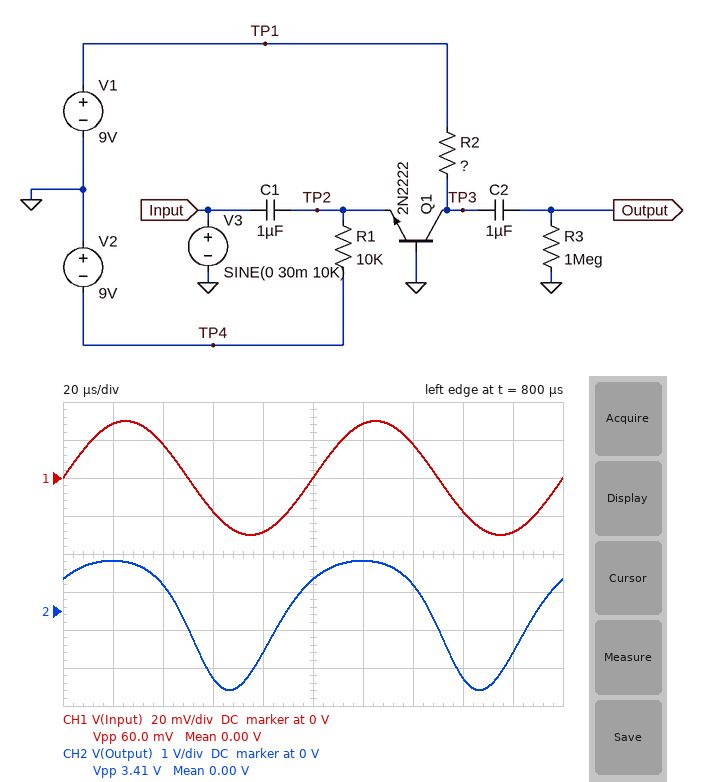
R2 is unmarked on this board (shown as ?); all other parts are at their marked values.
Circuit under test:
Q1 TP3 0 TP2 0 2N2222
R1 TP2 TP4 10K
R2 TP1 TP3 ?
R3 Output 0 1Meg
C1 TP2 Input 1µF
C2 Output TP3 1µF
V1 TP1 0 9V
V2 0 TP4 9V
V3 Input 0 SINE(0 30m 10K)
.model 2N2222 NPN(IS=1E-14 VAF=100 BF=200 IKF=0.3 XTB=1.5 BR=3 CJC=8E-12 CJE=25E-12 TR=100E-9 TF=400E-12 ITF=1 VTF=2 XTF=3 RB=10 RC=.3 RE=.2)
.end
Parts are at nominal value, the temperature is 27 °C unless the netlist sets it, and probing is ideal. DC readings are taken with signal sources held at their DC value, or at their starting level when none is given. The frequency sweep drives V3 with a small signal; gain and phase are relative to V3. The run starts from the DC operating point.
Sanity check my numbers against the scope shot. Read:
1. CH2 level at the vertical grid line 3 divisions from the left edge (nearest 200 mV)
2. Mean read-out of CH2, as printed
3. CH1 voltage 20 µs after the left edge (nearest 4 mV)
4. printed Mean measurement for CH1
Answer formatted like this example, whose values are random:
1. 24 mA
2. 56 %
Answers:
1. -1.8 V
2. 0.00 V
3. 28 mV
4. 0.00 V
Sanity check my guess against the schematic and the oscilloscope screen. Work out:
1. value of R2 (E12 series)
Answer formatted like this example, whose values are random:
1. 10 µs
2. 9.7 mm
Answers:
1. 2.2 kΩ
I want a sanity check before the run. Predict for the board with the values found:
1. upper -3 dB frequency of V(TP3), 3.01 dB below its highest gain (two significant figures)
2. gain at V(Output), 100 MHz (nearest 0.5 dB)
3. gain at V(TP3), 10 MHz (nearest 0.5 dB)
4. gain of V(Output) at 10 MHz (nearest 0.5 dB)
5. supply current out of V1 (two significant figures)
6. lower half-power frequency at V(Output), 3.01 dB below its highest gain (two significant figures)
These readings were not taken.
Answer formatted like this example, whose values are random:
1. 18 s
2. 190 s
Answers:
1. 15 MHz
2. 19.5 dB
3. 35.0 dB
4. 35.0 dB
5. 830 µA
6. 5.0 kHz
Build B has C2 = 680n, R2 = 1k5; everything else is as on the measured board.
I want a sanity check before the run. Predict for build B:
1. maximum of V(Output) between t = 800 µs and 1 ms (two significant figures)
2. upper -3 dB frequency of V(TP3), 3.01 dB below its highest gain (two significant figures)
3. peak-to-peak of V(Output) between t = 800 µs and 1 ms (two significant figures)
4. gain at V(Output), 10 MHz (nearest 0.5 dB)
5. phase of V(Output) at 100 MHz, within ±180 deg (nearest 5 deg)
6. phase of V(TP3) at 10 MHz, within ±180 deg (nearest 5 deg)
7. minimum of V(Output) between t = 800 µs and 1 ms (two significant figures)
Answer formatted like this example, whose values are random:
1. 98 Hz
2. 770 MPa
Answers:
1. 900 mV
2. 22 MHz
3. 2.3 V
4. 32.5 dB
5. -90 deg
6. -25 deg
7. -1.4 V
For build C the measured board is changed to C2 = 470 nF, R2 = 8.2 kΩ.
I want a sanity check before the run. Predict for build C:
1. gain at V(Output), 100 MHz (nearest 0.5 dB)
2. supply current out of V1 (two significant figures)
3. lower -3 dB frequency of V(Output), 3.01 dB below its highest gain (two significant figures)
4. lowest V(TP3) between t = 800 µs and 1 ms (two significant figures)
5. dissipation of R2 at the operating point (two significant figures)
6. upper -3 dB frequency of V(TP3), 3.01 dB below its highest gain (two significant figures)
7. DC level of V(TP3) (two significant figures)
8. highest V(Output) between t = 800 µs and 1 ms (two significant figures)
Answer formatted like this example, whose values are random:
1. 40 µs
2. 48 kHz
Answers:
1. 17.0 dB
2. 830 µA
3. 4.8 kHz
4. -650 mV
5. 5.7 mW
6. 3.1 MHz
7. 2.2 V
8. 4.5 V
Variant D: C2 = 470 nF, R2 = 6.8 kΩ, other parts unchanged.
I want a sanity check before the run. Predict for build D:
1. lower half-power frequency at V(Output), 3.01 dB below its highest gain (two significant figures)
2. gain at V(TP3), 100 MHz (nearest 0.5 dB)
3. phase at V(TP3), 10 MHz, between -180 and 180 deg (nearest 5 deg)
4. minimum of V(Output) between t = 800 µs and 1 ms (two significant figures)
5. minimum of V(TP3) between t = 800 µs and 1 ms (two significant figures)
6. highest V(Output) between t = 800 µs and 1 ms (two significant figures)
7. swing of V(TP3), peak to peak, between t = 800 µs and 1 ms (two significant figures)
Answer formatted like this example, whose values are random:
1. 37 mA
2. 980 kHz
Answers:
1. 4.8 kHz
2. 18.0 dB
3. -70 deg
4. -4.0 V
5. -630 mV
6. 3.9 V
7. 7.9 V
